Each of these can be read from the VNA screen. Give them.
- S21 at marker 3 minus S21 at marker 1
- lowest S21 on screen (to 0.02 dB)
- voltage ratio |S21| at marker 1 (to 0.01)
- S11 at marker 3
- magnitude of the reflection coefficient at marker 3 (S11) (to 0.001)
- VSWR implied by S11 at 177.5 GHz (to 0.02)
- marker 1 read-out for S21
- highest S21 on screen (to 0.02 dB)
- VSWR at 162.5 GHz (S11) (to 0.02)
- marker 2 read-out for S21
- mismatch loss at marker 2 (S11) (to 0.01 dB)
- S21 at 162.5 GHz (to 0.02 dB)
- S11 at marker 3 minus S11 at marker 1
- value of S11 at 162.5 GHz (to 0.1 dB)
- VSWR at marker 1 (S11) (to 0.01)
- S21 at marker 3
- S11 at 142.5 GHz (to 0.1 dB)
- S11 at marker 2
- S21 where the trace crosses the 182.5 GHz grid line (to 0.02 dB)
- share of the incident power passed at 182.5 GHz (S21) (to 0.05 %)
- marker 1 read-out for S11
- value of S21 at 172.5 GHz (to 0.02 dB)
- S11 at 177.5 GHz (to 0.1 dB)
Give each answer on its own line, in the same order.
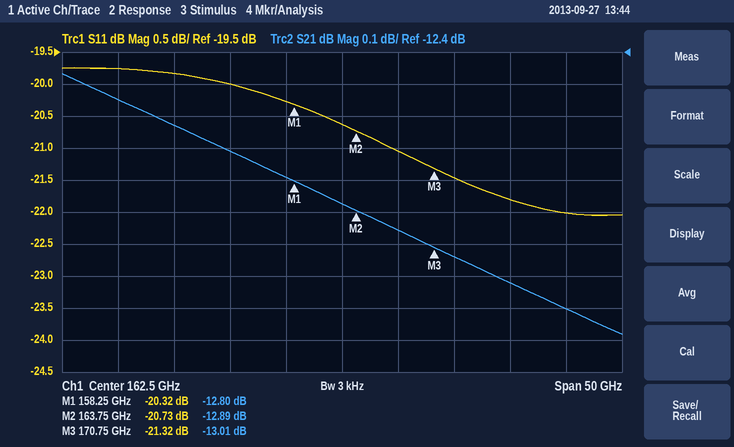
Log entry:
-0.21 dB
-13.28 dB
0.23
-21.32 dB
0.086
1.18
-12.80 dB
-12.46 dB
1.20
-12.89 dB
0.04 dB
-12.88 dB
-1.00 dB
-20.6 dB
1.21
-13.01 dB
-19.8 dB
-20.73 dB
-13.20 dB
4.80 %
-20.32 dB
-13.04 dB
-21.8 dB
